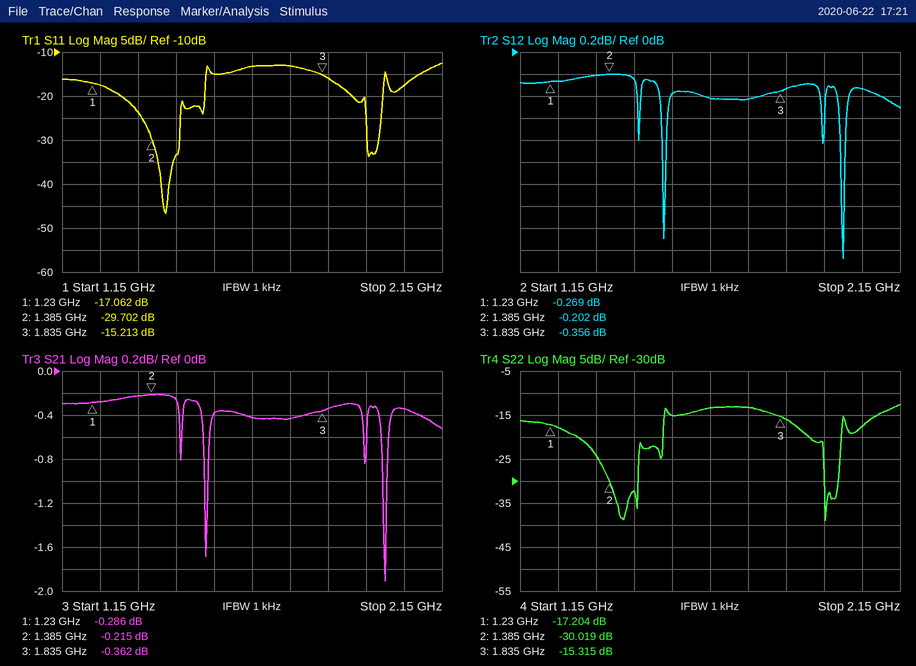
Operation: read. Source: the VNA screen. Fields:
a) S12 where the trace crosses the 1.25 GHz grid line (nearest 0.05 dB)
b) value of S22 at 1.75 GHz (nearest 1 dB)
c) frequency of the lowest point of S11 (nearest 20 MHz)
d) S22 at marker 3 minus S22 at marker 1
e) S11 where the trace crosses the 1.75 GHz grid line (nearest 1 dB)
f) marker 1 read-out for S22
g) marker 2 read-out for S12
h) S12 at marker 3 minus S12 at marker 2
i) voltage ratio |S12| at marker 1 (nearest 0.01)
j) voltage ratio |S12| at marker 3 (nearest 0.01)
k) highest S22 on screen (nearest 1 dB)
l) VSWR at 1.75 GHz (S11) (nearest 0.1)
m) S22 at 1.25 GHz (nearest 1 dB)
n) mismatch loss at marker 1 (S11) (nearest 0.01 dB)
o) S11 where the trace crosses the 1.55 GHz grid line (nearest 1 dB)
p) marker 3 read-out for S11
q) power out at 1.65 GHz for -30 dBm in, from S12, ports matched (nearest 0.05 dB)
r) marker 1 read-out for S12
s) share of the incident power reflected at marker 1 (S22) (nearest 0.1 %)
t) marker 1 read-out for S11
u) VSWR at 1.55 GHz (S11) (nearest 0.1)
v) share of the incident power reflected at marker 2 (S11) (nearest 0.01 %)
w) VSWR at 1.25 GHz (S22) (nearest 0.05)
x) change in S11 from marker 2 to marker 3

-0.25 dB
-13 dB
1.42 GHz
1.889 dB
-13 dB
-17.204 dB
-0.202 dB
-0.154 dB
0.97
0.96
-13 dB
1.6
-18 dB
0.09 dB
-15 dB
-15.213 dB
-30.40 dBm
-0.269 dB
1.9 %
-17.062 dB
1.4
0.11 %
1.30
14.489 dB
